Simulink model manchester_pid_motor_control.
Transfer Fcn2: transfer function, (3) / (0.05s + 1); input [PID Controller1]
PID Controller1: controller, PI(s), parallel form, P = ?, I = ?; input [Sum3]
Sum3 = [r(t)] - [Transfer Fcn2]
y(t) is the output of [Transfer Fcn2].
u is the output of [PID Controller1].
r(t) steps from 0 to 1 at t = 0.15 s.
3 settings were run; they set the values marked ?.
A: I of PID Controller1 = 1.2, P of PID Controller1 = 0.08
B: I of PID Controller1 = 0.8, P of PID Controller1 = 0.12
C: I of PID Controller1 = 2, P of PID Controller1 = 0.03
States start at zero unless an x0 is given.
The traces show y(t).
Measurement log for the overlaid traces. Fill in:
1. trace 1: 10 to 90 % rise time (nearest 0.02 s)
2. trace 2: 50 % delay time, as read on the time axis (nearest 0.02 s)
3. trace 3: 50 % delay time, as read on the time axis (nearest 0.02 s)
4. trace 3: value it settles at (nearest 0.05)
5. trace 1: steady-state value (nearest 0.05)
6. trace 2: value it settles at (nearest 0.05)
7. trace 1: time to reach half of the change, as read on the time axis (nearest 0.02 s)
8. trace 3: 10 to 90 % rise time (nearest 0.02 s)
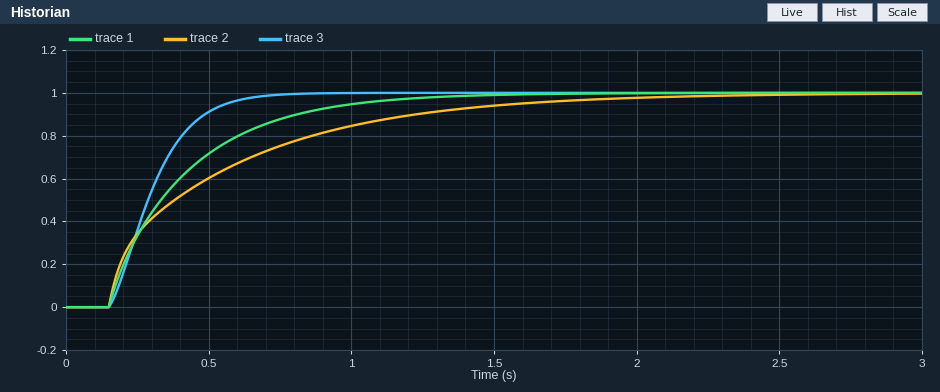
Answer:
0.64 s
0.38 s
0.28 s
1.00
1.00
1.00
0.34 s
0.30 s
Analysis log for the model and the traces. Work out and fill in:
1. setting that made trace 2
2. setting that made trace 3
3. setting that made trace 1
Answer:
B
C
A
